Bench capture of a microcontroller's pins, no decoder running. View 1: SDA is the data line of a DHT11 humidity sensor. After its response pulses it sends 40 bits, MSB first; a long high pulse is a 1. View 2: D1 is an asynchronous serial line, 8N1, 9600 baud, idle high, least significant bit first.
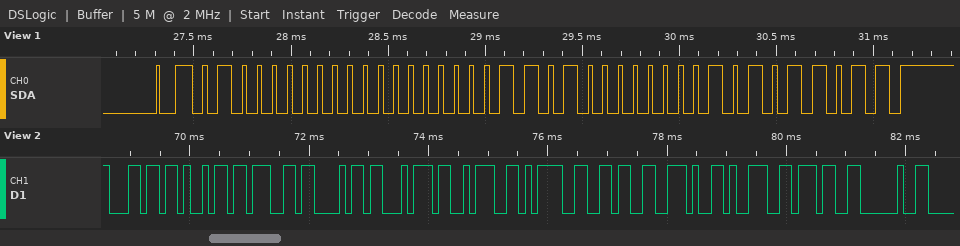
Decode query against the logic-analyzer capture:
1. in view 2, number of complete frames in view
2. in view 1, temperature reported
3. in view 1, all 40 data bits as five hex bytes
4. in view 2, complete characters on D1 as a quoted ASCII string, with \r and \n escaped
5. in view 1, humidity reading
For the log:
12
26.1 °C
40 00 1A 01 5B
"light:=6.97 "
64 %
